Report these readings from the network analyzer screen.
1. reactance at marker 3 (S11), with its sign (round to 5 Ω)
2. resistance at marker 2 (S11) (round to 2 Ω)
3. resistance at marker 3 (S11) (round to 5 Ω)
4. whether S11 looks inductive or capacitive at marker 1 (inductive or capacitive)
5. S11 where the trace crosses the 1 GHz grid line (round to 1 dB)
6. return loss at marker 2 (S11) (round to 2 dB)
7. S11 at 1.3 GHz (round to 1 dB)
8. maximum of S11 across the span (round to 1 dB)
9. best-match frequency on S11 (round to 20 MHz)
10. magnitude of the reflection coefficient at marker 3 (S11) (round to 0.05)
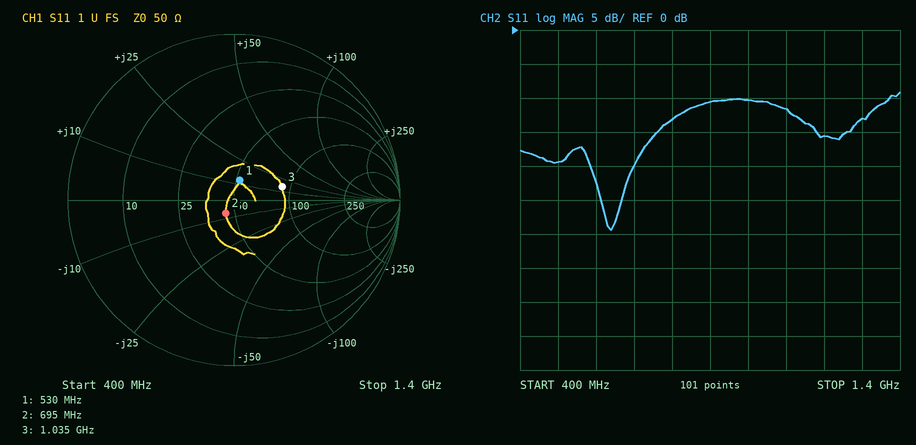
+15 Ω
44 Ω
90 Ω
inductive
-10 dB
20 dB
-13 dB
-9 dB
640 MHz
0.30
